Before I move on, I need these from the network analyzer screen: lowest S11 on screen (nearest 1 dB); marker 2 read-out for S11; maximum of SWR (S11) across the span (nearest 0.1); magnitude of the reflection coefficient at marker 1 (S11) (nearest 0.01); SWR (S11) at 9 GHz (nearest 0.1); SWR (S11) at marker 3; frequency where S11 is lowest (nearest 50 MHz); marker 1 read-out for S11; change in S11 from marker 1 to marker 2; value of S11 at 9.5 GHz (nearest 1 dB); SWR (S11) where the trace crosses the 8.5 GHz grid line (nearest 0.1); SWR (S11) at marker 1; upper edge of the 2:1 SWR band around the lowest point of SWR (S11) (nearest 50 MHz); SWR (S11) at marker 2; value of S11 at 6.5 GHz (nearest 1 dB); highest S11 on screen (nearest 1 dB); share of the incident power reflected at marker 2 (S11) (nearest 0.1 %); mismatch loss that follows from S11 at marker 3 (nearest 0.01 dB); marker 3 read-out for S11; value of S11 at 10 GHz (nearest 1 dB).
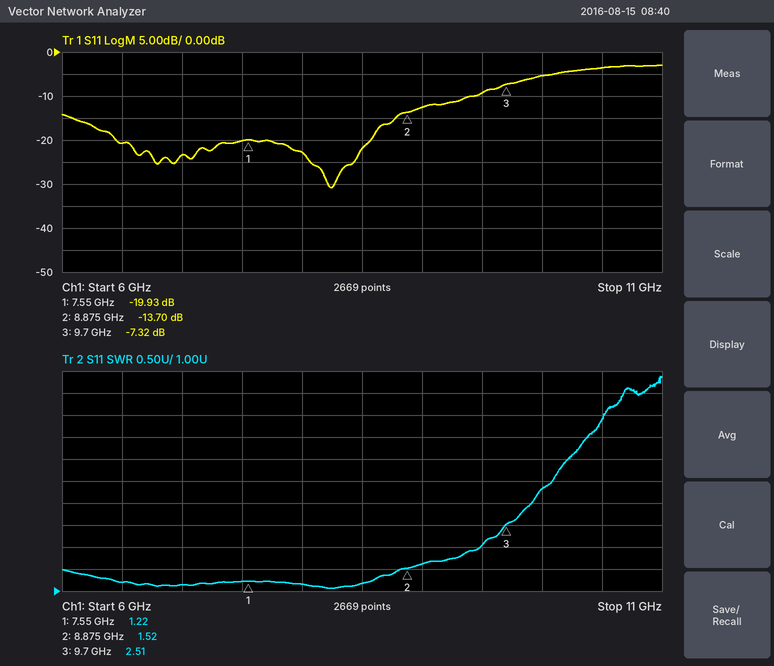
-31 dB
-13.70 dB
5.9
0.10
1.6
2.51
8.25 GHz
-19.93 dB
6.23 dB
-9 dB
1.2
1.22
9.50 GHz
1.52
-21 dB
-3 dB
4.3 %
0.89 dB
-7.32 dB
-5 dB
